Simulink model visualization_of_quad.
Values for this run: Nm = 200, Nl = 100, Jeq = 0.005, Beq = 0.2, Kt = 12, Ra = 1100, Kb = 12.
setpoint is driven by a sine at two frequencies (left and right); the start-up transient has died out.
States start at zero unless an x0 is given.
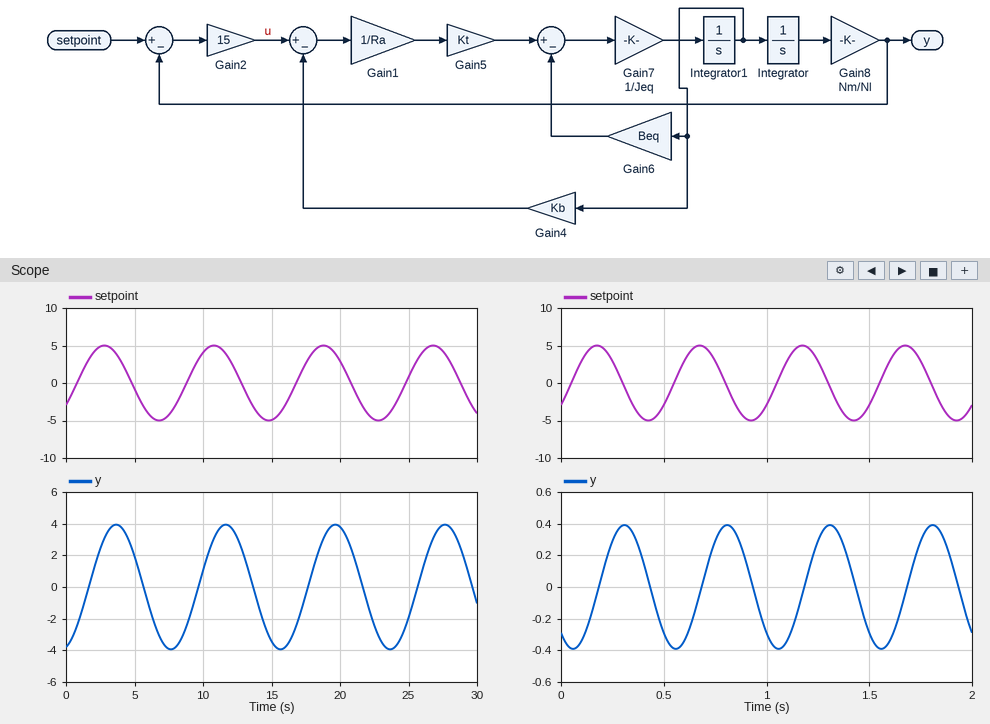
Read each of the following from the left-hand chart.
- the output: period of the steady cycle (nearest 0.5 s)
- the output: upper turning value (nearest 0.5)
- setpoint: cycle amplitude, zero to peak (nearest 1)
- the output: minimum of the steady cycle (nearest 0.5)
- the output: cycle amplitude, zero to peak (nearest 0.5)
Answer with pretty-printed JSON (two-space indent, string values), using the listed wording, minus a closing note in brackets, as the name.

{
  "the output: period of the steady cycle": "8.0 s",
  "the output: upper turning value": "4.0",
  "setpoint: cycle amplitude, zero to peak": "5",
  "the output: minimum of the steady cycle": "-4.0",
  "the output: cycle amplitude, zero to peak": "4.0"
}
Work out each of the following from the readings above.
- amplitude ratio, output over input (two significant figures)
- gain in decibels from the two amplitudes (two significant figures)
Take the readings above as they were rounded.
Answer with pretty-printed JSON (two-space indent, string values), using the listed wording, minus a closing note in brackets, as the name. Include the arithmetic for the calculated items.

{
  "amplitude ratio, output over input": "4 / 5 = 0.80",
  "gain in decibels from the two amplitudes": "20 log10(4 / 5) = -1.9 dB"
}
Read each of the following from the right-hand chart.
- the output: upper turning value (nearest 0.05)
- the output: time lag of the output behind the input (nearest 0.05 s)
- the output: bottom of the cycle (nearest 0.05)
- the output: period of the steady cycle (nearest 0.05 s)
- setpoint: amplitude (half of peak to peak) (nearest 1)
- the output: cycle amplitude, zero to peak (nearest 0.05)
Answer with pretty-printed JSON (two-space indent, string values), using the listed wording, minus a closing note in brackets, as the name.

{
  "the output: upper turning value": "0.40",
  "the output: time lag of the output behind the input": "0.15 s",
  "the output: bottom of the cycle": "-0.40",
  "the output: period of the steady cycle": "0.50 s",
  "setpoint: amplitude (half of peak to peak)": "5",
  "the output: cycle amplitude, zero to peak": "0.40"
}
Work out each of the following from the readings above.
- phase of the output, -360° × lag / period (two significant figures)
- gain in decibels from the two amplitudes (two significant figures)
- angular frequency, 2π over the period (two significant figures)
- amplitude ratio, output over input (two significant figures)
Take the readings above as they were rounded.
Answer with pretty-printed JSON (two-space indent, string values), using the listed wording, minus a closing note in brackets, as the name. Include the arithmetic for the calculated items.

{
  "phase of the output, -360° × lag / period": "-360 × 0.15 / 0.5 = -110°",
  "gain in decibels from the two amplitudes": "20 log10(0.4 / 5) = -22 dB",
  "angular frequency, 2π over the period": "2π / 0.5 = 13 rad/s",
  "amplitude ratio, output over input": "0.4 / 5 = 0.080"
}
